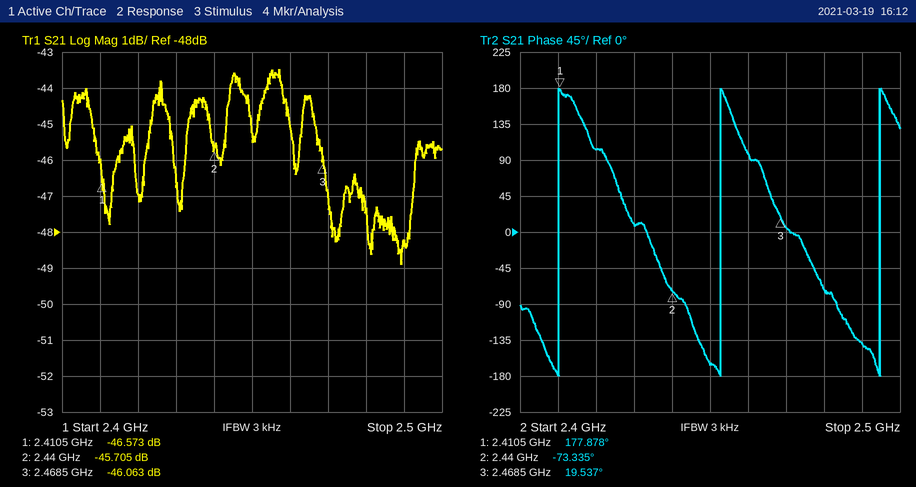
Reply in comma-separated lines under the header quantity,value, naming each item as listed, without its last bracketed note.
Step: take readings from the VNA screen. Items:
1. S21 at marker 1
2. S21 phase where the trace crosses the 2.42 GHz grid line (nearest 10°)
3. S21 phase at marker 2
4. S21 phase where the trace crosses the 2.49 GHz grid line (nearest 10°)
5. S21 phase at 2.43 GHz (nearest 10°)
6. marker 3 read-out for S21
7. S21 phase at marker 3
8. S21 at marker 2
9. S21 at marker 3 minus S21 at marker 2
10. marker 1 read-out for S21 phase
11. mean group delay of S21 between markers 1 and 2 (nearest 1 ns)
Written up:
quantity,value
S21 at marker 1,-46.573 dB
S21 phase where the trace crosses the 2.42 GHz grid line,100°
S21 phase at marker 2,-73.335°
S21 phase where the trace crosses the 2.49 GHz grid line,-140°
S21 phase at 2.43 GHz,10°
marker 3 read-out for S21,-46.063 dB
S21 phase at marker 3,19.537°
S21 at marker 2,-45.705 dB
S21 at marker 3 minus S21 at marker 2,-0.358 dB
marker 1 read-out for S21 phase,177.878°
mean group delay of S21 between markers 1 and 2,24 ns
